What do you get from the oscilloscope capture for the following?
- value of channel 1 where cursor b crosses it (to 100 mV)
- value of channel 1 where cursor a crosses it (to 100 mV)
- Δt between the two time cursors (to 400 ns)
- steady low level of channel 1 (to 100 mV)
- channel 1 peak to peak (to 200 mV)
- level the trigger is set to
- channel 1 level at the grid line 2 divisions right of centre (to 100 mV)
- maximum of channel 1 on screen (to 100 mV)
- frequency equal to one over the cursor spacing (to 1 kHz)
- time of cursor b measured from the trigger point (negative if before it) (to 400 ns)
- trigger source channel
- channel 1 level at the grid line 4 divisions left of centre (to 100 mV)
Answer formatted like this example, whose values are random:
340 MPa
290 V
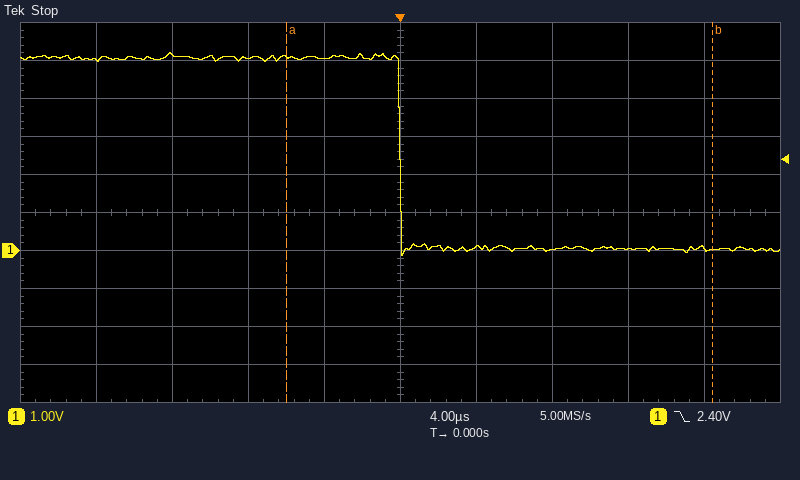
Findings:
0.0 V
5.1 V
22.4 µs
100 mV
5.4 V
2.40 V
0.0 V
5.2 V
45 kHz
+16.4 µs
channel 1
5.0 V
